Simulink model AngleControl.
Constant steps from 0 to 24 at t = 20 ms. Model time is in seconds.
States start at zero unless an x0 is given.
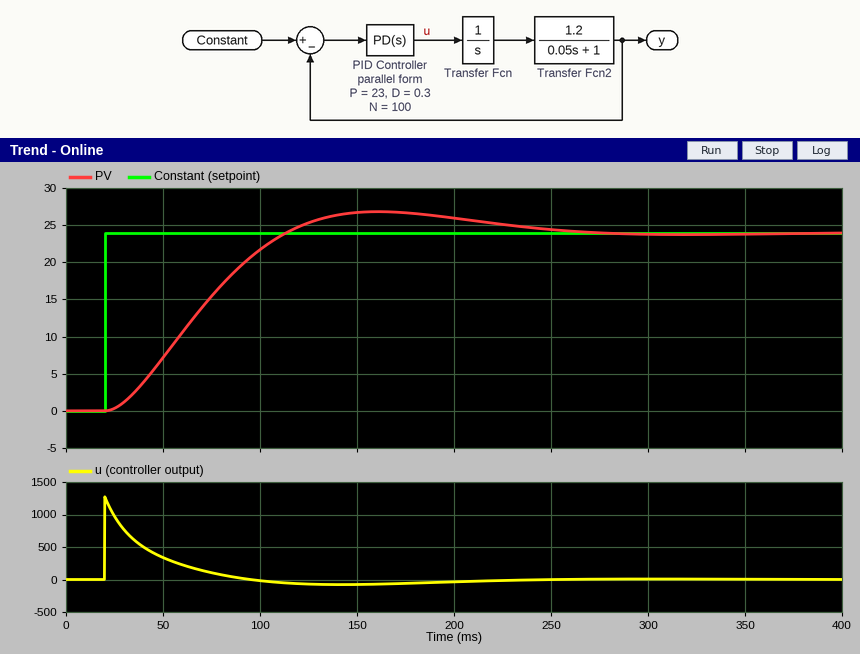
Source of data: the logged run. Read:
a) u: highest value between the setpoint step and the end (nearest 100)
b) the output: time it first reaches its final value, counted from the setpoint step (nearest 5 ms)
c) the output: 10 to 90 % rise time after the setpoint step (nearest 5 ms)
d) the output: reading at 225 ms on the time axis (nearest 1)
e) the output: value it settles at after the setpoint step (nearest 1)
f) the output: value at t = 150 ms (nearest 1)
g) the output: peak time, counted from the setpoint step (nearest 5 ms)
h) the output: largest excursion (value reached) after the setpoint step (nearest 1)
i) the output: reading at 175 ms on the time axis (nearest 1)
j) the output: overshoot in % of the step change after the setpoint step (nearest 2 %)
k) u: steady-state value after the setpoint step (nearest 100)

1300
95 ms
65 ms
25
24
27
140 ms
27
27
12 %
0
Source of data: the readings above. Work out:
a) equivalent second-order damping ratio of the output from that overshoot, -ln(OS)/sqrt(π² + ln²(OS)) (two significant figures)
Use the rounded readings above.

0.56
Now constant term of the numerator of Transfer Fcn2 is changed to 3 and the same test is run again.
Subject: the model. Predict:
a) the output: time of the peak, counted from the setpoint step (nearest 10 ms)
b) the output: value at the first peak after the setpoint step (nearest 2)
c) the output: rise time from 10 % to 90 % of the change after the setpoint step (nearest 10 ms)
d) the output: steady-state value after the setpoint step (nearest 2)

70 ms
30
30 ms
24
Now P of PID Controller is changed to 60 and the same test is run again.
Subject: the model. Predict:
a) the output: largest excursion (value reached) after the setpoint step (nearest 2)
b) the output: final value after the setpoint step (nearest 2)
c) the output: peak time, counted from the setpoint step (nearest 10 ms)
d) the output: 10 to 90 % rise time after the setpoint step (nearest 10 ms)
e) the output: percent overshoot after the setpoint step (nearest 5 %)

32
24
80 ms
30 ms
35 %
